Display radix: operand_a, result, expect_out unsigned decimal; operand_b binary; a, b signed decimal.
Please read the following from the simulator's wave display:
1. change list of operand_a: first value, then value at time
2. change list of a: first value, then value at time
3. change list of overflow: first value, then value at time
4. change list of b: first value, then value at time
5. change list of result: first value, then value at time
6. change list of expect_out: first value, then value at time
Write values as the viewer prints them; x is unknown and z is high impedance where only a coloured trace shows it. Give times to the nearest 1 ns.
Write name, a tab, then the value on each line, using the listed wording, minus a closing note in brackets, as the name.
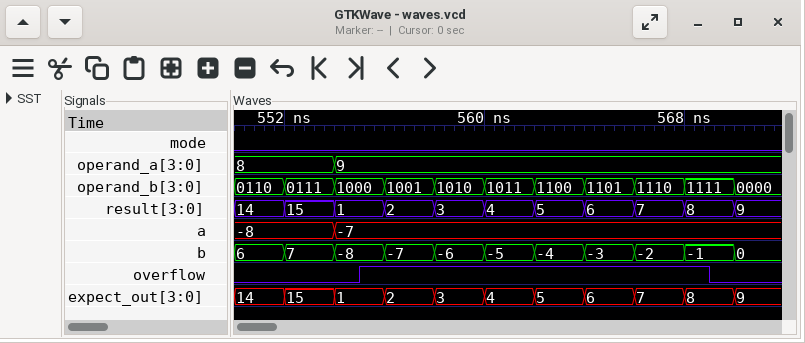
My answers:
change list of operand_a: first value, then value at time	8, 9 at 554 ns
change list of a: first value, then value at time	-8, -7 at 554 ns
change list of overflow: first value, then value at time	0, 1 at 555 ns, 0 at 569 ns
change list of b: first value, then value at time	6, 7 at 552 ns, -8 at 554 ns, -7 at 556 ns, -6 at 558 ns, -5 at 560 ns, -4 at 562 ns, -3 at 564 ns, -2 at 566 ns, -1 at 568 ns, 0 at 570 ns
change list of result: first value, then value at time	14, 15 at 552 ns, 1 at 554 ns, 2 at 556 ns, 3 at 558 ns, 4 at 560 ns, 5 at 562 ns, 6 at 564 ns, 7 at 566 ns, 8 at 568 ns, 9 at 570 ns
change list of expect_out: first value, then value at time	14, 15 at 552 ns, 1 at 554 ns, 2 at 556 ns, 3 at 558 ns, 4 at 560 ns, 5 at 562 ns, 6 at 564 ns, 7 at 566 ns, 8 at 568 ns, 9 at 570 ns
